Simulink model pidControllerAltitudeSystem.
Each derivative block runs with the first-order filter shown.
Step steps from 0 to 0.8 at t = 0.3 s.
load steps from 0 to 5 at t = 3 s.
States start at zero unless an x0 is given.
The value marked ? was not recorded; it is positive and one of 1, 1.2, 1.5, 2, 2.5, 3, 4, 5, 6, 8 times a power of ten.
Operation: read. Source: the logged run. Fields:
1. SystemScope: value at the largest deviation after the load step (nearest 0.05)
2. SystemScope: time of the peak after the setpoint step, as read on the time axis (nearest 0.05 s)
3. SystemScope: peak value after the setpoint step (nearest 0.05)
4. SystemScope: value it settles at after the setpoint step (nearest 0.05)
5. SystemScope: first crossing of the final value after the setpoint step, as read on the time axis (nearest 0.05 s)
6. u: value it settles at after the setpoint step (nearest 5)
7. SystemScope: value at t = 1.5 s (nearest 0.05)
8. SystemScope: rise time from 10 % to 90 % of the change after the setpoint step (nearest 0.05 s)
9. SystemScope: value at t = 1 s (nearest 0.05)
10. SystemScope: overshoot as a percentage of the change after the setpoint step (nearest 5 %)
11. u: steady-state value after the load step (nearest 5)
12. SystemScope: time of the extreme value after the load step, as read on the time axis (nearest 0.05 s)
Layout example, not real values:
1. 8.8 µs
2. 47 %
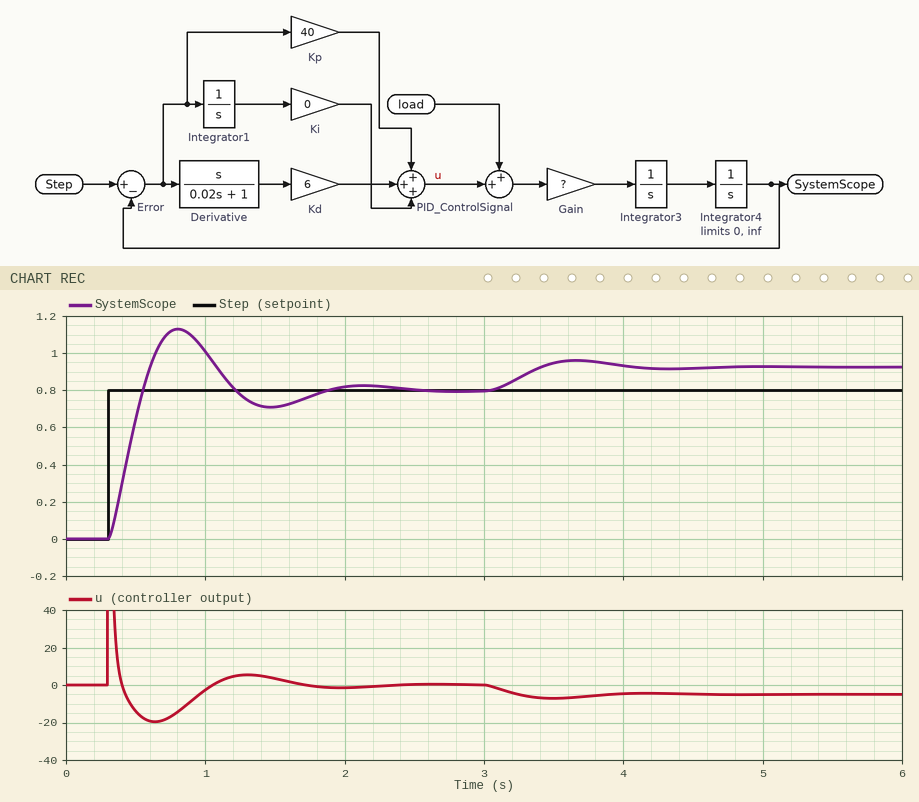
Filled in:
1. 0.95
2. 0.80 s
3. 1.15
4. 0.80
5. 0.55 s
6. 0
7. 0.70
8. 0.20 s
9. 1.00
10. 40 %
11. -5
12. 3.65 s
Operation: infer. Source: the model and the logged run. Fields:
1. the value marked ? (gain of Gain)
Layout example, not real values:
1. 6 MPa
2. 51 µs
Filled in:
1. 0.6
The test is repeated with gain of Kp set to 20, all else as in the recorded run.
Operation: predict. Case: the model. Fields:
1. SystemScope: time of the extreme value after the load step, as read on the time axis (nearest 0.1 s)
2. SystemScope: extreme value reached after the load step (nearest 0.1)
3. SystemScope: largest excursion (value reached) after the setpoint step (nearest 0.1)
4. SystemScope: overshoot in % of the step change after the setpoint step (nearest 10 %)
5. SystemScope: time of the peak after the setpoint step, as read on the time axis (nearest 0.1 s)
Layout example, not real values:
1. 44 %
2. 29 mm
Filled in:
1. 4.0 s
2. 1.1
3. 1.0
4. 30 %
5. 1.0 s
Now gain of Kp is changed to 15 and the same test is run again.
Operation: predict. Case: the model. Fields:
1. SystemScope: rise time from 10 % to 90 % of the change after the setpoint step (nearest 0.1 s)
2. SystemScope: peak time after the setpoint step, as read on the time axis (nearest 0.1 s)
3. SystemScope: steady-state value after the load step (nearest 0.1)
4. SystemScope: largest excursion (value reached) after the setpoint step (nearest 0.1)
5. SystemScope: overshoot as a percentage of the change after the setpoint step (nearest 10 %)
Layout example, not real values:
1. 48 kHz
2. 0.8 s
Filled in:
1. 0.3 s
2. 1.0 s
3. 1.1
4. 1.0
5. 30 %
